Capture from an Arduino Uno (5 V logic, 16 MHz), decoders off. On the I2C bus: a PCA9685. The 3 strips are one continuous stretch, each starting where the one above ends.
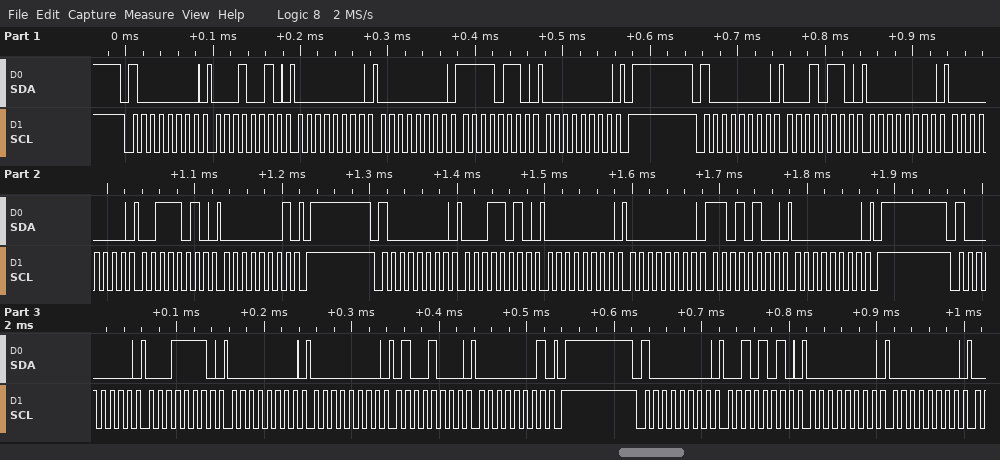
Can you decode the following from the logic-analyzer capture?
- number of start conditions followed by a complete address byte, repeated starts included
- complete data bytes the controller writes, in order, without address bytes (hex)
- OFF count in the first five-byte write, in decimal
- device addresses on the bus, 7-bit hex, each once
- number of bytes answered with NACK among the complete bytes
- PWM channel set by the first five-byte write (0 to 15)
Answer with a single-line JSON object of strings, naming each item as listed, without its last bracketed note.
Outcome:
{"number of start conditions followed by a complete address byte, repeated starts included": "5", "complete data bytes the controller writes, in order, without address bytes": "12 00 00 F6 00 16 00 00 3A 01 1A 00 00 D4 00 1E 00 00 48 01 2A 00 00", "OFF count in the first five-byte write, in decimal": "246", "device addresses on the bus, 7-bit hex, each once": "0x40", "number of bytes answered with NACK among the complete bytes": "0", "PWM channel set by the first five-byte write": "3"}
